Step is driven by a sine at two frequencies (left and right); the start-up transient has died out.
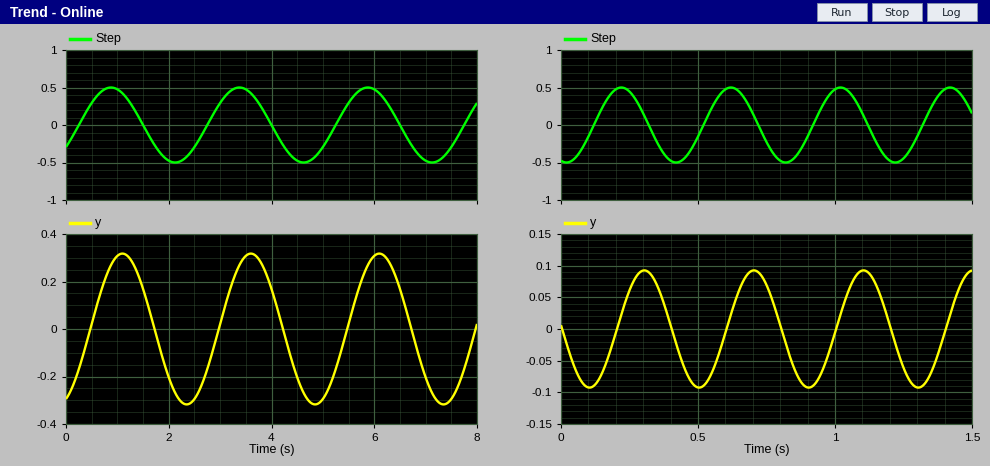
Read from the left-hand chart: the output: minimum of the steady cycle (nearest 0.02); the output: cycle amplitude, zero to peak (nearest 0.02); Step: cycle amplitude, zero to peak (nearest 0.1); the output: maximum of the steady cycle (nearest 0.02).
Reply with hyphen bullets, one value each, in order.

- -0.32
- 0.32
- 0.5
- 0.32
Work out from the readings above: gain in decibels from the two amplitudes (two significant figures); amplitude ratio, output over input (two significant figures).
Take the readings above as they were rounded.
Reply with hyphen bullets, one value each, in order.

- -3.9 dB
- 0.64
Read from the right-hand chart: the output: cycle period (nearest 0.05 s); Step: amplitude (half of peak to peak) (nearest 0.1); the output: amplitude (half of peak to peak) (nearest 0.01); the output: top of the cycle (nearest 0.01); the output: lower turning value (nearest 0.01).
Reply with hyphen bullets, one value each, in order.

- 0.40 s
- 0.5
- 0.09
- 0.09
- -0.09
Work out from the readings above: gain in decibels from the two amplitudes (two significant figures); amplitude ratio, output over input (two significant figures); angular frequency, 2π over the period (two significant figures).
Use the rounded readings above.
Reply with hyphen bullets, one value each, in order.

- -15 dB
- 0.18
- 16 rad/s
